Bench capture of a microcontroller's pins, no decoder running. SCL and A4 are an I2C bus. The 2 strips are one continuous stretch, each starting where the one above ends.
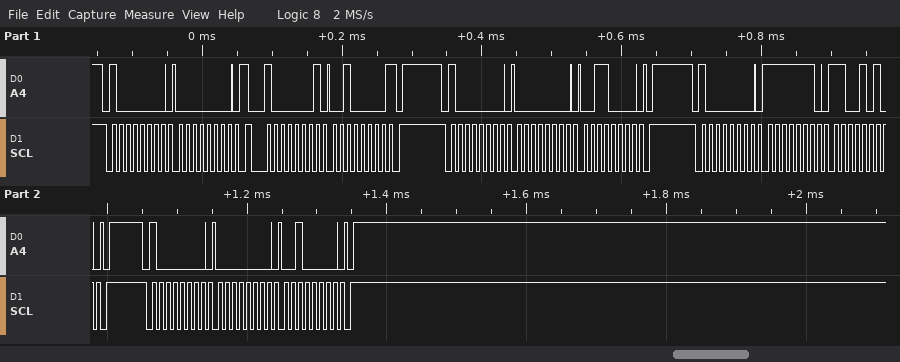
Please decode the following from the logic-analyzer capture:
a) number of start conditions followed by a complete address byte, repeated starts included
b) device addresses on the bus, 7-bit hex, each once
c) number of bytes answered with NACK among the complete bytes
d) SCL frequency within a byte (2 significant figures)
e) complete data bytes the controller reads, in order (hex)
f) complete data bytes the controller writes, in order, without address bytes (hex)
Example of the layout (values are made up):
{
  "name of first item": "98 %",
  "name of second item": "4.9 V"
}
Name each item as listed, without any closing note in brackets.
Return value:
{
  "number of start conditions followed by a complete address byte, repeated starts included": "5",
  "device addresses on the bus, 7-bit hex, each once": "0x40",
  "number of bytes answered with NACK among the complete bytes": "1",
  "SCL frequency within a byte": "100 kHz",
  "complete data bytes the controller reads, in order": "20",
  "complete data bytes the controller writes, in order, without address bytes": "00 00 30 FE CA 00 20"
}
